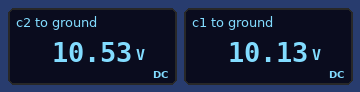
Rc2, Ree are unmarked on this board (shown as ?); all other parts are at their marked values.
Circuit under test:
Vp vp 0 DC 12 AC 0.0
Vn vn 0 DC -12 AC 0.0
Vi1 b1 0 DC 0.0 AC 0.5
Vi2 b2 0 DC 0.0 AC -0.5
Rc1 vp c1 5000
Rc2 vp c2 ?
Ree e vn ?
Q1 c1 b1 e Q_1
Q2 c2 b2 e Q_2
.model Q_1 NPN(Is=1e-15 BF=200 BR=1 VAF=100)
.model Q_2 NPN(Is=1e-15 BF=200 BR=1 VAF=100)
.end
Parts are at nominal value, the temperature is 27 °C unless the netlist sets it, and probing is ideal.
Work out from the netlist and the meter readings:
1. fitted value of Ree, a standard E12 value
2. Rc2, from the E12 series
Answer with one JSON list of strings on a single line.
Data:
["15 kΩ", "3.9 kΩ"]
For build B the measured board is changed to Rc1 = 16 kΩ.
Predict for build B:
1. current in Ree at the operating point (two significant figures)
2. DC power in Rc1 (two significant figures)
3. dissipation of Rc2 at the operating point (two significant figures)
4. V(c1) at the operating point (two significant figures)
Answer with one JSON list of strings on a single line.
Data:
["750 µA", "2.2 mW", "570 µW", "6.1 V"]
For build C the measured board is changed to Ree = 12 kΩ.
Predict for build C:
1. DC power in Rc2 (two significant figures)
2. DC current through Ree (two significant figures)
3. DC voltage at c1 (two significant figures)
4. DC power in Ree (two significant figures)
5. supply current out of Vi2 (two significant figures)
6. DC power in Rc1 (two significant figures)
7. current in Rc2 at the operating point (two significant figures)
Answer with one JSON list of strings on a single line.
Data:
["860 µW", "940 µA", "9.7 V", "11 mW", "2.1 µA", "1.1 mW", "470 µA"]
